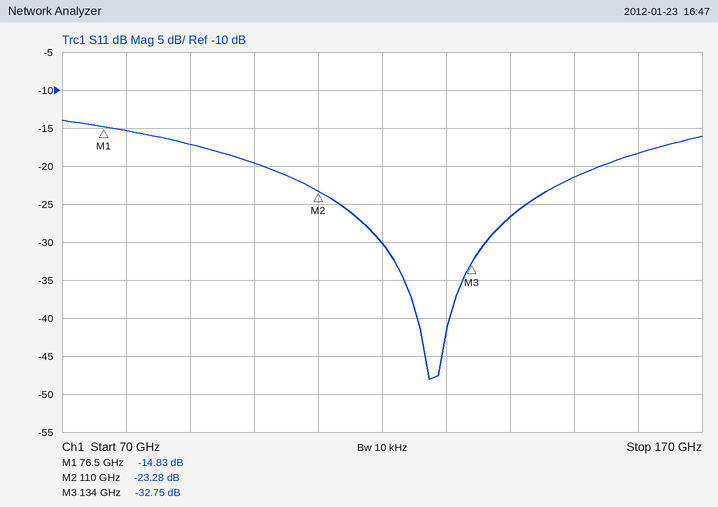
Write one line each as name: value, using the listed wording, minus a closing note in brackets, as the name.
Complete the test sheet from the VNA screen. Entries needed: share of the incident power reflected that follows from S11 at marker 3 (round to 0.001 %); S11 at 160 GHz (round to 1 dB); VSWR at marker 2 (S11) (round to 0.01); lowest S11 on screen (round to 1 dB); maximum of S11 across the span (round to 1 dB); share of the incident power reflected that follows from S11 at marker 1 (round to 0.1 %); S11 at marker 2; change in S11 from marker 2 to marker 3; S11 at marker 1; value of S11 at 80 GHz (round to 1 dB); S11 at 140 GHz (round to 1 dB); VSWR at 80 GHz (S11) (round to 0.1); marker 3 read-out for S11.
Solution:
share of the incident power reflected that follows from S11 at marker 3: 0.053 %
S11 at 160 GHz: -18 dB
VSWR at marker 2 (S11): 1.15
lowest S11 on screen: -48 dB
maximum of S11 across the span: -14 dB
share of the incident power reflected that follows from S11 at marker 1: 3.3 %
S11 at marker 2: -23.28 dB
change in S11 from marker 2 to marker 3: -9.47 dB
S11 at marker 1: -14.83 dB
value of S11 at 80 GHz: -15 dB
S11 at 140 GHz: -27 dB
VSWR at 80 GHz (S11): 1.4
marker 3 read-out for S11: -32.75 dB
